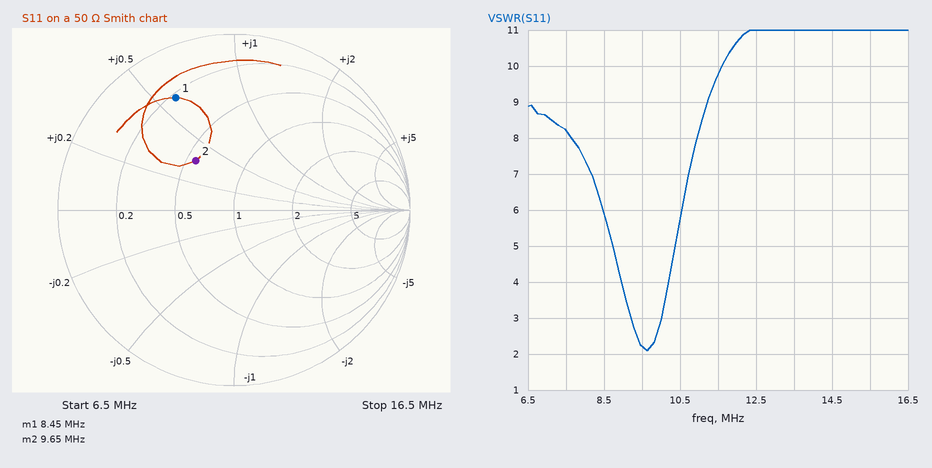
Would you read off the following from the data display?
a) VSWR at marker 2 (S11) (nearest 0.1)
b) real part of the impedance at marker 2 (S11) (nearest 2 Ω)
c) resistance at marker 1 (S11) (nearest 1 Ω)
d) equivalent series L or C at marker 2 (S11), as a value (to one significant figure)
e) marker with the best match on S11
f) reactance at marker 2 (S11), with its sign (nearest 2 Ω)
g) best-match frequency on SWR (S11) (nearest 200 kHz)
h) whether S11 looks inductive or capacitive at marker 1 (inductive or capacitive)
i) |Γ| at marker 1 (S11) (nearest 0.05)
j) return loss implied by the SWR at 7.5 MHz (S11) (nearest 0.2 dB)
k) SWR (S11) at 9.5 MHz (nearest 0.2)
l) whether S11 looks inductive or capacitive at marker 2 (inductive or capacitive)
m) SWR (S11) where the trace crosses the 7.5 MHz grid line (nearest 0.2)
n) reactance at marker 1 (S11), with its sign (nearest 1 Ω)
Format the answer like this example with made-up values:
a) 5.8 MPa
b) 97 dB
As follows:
a) 2.1
b) 28 Ω
c) 11 Ω
d) 300 nH
e) marker 2
f) +18 Ω
g) 9.6 MHz
h) inductive
i) 0.70
j) 2.2 dB
k) 2.2
l) inductive
m) 8.2
n) +29 Ω
